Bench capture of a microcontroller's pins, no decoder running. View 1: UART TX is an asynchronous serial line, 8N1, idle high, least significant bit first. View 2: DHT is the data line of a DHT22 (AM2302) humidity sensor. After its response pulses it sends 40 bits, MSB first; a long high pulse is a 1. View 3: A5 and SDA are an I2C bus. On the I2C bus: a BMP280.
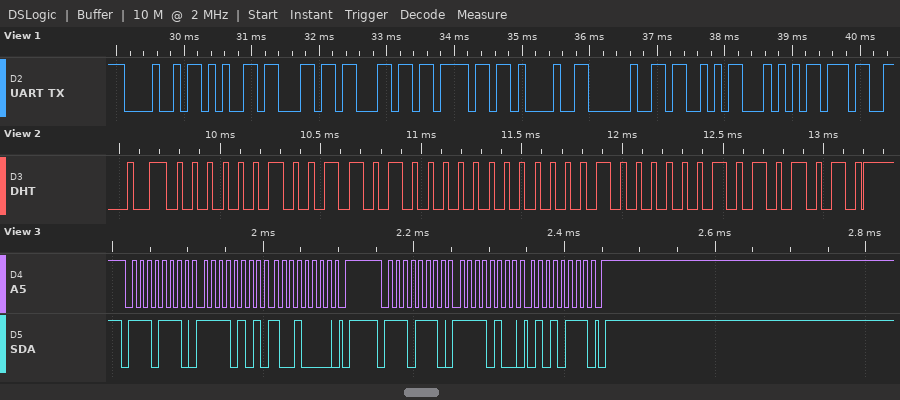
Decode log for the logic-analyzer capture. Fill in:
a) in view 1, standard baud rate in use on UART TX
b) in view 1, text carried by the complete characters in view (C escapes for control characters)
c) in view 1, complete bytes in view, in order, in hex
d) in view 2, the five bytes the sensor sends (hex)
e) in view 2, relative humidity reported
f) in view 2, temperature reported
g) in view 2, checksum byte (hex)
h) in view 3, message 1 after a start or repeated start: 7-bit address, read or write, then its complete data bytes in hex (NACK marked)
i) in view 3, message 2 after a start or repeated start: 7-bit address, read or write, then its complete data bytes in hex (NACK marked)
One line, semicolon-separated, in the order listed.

9600 baud; "Hello! ST7"; 48 65 6C 6C 6F 21 20 53 54 37; 02 68 00 40 AA; 61.6 %; 6.4 °C; 0xAA; 0x77 write: F5 90; 0x77 write: F4 57
